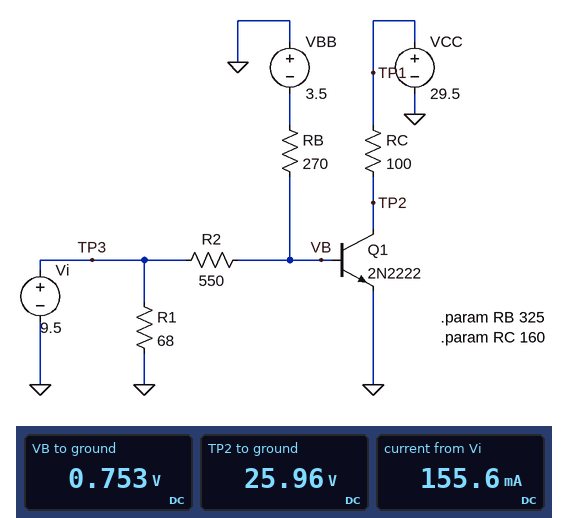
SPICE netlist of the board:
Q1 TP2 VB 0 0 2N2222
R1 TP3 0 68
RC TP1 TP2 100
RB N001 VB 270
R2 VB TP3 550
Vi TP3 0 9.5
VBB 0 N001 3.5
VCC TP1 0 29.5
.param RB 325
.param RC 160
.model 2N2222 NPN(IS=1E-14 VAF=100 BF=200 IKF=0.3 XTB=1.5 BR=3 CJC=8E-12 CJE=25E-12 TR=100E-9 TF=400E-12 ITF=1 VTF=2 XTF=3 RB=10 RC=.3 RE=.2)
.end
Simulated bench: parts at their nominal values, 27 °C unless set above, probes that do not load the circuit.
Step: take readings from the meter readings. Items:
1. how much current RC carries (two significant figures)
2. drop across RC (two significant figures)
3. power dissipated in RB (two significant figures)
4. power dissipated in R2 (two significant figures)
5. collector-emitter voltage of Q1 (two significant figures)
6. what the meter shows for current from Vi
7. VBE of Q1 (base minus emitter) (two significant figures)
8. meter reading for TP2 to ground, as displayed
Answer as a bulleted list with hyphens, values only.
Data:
- 35 mA
- 3.5 V
- 67 mW
- 140 mW
- 26 V
- 155.6 mA
- 750 mV
- 25.96 V
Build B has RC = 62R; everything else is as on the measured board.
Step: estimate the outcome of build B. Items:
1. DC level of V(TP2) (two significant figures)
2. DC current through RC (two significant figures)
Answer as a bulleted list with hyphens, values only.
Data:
- 27 V
- 36 mA
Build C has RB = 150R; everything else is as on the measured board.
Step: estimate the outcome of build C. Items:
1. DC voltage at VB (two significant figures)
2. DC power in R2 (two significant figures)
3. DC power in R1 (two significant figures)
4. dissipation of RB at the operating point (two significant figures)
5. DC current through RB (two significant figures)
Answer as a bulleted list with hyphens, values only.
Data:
- -710 mV
- 190 mW
- 1.3 W
- 52 mW
- 19 mA
